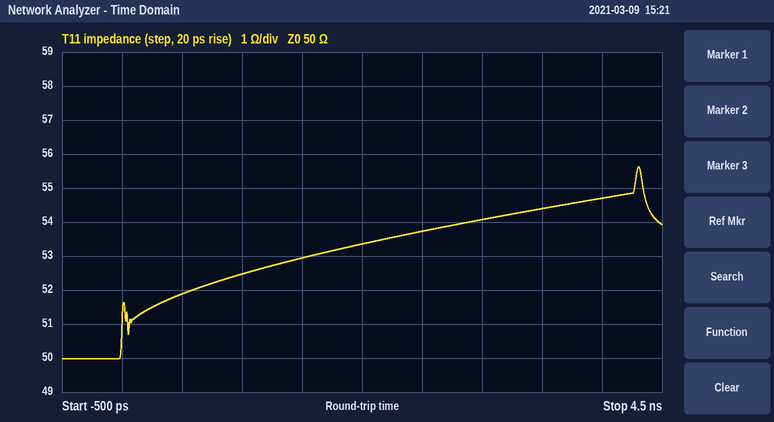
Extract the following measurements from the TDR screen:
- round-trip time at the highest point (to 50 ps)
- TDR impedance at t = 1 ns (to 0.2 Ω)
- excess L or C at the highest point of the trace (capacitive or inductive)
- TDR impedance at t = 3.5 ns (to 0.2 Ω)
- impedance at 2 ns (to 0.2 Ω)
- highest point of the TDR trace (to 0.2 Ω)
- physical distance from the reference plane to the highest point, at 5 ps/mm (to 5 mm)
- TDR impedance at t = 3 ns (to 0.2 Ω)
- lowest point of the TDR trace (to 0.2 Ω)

4.30 ns
52.4 Ω
inductive
54.4 Ω
53.4 Ω
55.6 Ω
430 mm
54.0 Ω
50.0 Ω
